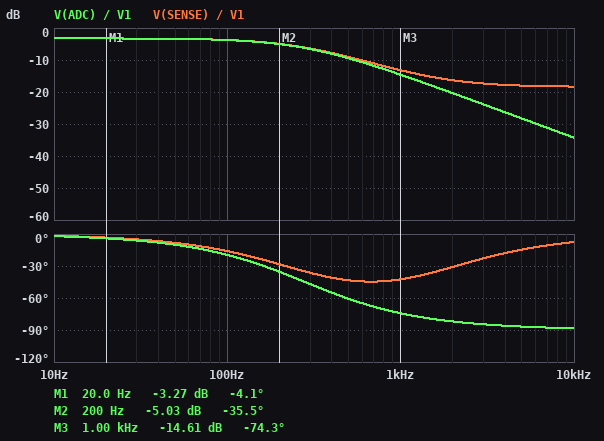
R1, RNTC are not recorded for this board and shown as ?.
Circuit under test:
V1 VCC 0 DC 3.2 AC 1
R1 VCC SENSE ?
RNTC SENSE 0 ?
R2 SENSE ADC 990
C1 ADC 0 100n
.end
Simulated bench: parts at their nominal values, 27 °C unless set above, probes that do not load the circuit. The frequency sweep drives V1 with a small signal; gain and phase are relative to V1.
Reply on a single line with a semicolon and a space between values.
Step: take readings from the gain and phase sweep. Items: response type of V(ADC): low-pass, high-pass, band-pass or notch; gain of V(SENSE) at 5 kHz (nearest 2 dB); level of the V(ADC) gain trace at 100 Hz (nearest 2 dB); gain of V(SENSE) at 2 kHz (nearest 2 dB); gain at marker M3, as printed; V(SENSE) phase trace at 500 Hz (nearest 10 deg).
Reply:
low-pass; -18 dB; -4 dB; -16 dB; -14.61 dB; -40 deg
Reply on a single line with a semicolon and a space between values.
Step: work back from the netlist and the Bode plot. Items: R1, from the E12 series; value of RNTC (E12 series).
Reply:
6.8 kΩ; 15 kΩ
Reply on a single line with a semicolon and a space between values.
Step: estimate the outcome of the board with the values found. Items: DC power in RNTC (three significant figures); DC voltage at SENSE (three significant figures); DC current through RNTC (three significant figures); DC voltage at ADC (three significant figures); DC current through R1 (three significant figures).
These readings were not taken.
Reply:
323 µW; 2.20 V; 147 µA; 2.20 V; 147 µA
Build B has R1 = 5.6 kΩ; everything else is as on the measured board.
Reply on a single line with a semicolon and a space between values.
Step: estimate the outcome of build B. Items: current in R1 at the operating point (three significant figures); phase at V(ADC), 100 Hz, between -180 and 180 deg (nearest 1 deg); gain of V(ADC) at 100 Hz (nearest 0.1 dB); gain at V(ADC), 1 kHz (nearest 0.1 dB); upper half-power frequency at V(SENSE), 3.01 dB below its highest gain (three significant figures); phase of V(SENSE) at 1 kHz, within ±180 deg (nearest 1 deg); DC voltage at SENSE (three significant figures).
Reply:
155 µA; -18 deg; -3.2 dB; -13.2 dB; 327 Hz; -41 deg; 2.33 V
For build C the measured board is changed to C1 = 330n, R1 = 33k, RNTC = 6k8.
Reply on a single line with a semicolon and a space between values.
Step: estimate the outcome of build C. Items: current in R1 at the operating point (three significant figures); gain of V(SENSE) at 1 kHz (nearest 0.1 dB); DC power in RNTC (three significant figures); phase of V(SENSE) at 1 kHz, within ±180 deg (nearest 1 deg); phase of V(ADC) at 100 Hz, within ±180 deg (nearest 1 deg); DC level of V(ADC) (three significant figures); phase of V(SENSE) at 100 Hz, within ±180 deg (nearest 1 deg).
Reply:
80.4 µA; -31.0 dB; 44.0 µW; -22 deg; -54 deg; 547 mV; -42 deg
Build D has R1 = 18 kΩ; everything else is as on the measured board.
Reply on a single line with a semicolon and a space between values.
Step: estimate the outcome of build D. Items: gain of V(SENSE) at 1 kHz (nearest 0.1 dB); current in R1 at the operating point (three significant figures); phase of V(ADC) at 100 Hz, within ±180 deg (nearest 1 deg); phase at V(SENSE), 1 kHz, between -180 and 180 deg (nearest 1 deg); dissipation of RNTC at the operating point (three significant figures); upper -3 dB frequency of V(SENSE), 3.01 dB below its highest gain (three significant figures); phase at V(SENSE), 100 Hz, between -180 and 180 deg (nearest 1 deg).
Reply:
-20.8 dB; 97.0 µA; -30 deg; -48 deg; 141 µW; 176 Hz; -26 deg
